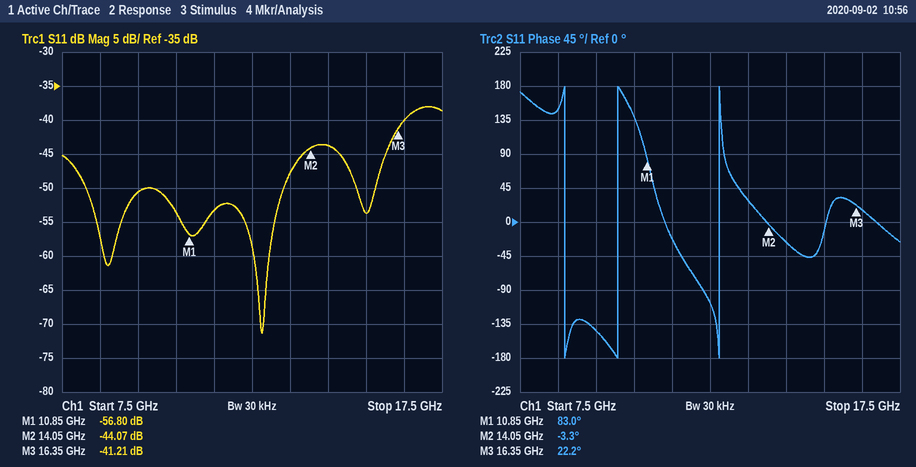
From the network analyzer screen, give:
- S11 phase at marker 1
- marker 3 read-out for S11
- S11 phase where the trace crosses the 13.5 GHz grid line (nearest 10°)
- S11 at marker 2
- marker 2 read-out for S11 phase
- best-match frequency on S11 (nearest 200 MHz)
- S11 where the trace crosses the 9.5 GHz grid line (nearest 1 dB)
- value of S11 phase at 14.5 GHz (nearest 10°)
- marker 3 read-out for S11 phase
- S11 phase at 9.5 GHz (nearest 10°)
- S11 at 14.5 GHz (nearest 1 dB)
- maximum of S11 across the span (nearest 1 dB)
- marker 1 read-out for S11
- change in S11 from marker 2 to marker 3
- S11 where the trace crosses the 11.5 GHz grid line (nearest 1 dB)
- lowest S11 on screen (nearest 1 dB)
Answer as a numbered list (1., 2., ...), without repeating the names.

1. 83.0°
2. -41.21 dB
3. 30°
4. -44.07 dB
5. -3.3°
6. 12.8 GHz
7. -51 dB
8. -30°
9. 22.2°
10. -140°
11. -44 dB
12. -38 dB
13. -56.80 dB
14. 2.86 dB
15. -53 dB
16. -71 dB
